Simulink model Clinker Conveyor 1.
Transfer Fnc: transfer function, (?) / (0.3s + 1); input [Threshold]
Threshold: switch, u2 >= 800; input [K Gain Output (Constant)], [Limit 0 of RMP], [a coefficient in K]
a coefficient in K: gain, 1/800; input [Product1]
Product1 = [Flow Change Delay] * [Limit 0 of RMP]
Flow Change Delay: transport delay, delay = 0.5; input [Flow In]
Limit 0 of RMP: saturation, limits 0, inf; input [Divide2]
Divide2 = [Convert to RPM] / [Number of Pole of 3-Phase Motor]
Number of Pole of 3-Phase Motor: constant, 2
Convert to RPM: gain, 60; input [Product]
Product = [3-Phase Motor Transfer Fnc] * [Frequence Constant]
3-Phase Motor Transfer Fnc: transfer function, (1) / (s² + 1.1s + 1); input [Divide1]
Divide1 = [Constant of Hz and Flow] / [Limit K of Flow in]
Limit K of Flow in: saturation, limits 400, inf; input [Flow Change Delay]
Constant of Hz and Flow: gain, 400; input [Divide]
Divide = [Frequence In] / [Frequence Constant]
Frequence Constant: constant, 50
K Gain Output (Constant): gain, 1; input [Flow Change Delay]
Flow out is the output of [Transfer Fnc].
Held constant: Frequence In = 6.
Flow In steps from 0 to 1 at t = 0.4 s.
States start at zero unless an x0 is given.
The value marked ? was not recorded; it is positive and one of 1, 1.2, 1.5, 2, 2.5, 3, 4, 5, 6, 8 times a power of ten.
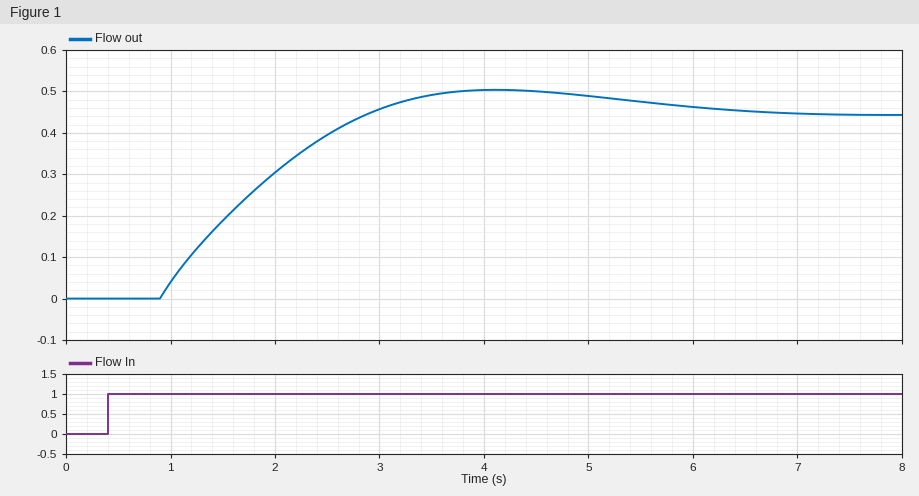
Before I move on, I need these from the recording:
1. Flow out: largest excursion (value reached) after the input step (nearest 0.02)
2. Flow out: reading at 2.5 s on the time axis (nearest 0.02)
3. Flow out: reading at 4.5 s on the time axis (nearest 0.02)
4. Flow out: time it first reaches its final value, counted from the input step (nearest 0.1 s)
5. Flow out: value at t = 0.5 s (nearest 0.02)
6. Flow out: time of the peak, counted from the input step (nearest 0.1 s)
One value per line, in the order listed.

0.50
0.40
0.50
2.5 s
0.00
3.7 s
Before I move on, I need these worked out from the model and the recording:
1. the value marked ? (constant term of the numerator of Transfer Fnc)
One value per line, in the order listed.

2
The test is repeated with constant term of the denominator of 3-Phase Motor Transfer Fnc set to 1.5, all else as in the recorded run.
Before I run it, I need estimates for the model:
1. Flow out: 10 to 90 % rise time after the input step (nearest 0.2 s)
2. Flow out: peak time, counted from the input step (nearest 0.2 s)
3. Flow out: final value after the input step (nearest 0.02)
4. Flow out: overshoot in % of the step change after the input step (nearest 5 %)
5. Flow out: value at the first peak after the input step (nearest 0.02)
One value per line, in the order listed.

1.0 s
2.8 s
0.30
20 %
0.36
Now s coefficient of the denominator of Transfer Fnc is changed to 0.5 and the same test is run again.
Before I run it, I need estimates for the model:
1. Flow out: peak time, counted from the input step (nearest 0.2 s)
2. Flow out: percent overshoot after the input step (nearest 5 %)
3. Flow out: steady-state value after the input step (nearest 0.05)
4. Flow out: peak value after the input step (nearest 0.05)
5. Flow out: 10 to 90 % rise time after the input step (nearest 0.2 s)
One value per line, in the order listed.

4.0 s
10 %
0.45
0.50
1.8 s
